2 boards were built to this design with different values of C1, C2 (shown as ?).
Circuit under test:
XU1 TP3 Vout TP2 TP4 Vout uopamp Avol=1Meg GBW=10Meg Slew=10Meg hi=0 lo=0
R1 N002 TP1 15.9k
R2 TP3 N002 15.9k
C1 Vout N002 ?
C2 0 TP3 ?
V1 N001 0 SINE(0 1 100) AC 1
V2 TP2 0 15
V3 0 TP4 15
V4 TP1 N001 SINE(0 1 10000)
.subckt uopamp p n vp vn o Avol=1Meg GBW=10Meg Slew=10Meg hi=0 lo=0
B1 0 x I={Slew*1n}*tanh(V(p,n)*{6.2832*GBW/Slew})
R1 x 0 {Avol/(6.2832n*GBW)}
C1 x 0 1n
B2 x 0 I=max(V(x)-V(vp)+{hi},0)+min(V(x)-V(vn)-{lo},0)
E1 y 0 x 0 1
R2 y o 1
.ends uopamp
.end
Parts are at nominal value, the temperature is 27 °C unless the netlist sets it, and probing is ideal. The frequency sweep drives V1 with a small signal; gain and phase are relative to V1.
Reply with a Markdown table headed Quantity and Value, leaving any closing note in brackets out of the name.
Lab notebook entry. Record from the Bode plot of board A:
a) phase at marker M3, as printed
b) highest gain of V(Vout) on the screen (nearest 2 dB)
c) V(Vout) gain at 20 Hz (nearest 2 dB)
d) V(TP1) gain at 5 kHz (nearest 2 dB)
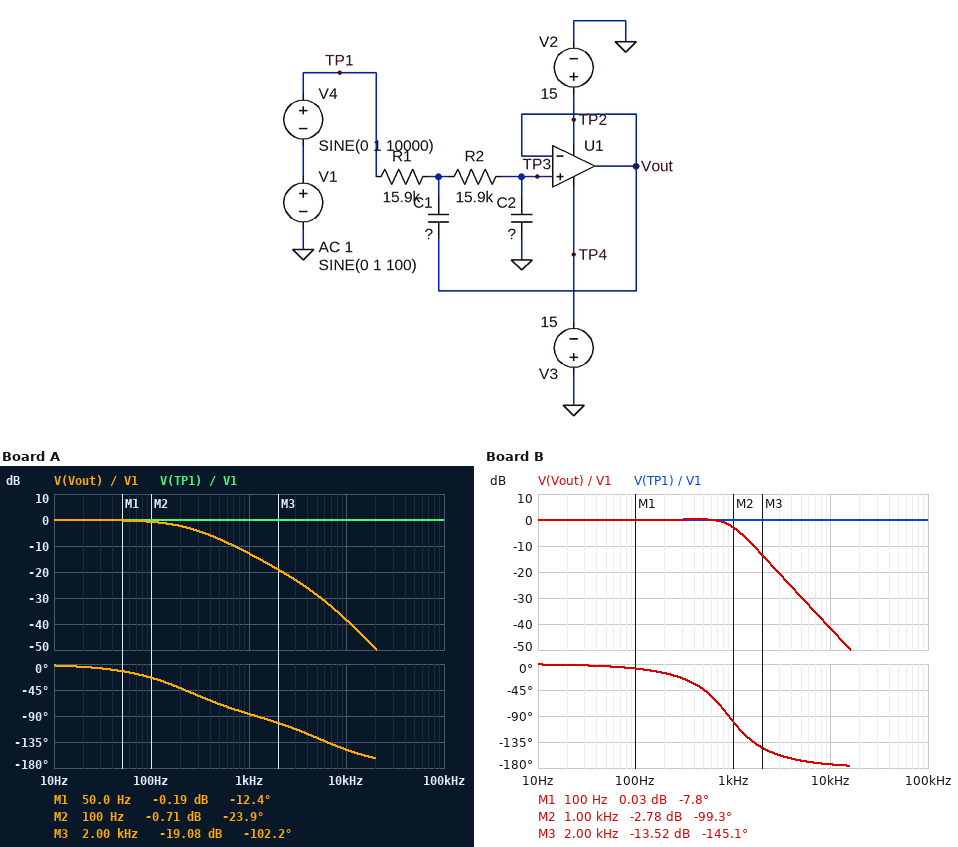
| Quantity | Value |
|---|---|
| phase at marker M3, as printed | -102.2 deg |
| highest gain of V(Vout) on the screen | 0 dB |
| V(Vout) gain at 20 Hz | 0 dB |
| V(TP1) gain at 5 kHz | 0 dB |
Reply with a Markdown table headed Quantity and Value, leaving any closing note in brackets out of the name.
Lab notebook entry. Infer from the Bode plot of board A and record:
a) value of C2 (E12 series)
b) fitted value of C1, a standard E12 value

| Quantity | Value |
|---|---|
| value of C2 | 22 nF |
| fitted value of C1, a standard E12 value | 3.3 nF |
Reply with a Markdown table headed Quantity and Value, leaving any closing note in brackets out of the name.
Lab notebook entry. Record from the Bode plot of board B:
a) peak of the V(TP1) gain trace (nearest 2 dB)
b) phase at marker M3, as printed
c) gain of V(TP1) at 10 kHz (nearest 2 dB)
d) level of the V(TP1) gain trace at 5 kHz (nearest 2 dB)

| Quantity | Value |
|---|---|
| peak of the V(TP1) gain trace | 0 dB |
| phase at marker M3, as printed | -145.1 deg |
| gain of V(TP1) at 10 kHz | 0 dB |
| level of the V(TP1) gain trace at 5 kHz | 0 dB |
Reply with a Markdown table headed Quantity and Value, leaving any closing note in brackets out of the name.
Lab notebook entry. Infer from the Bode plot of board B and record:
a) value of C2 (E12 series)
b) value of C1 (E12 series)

| Quantity | Value |
|---|---|
| value of C2 | 6.8 nF |
| value of C1 | 18 nF |
